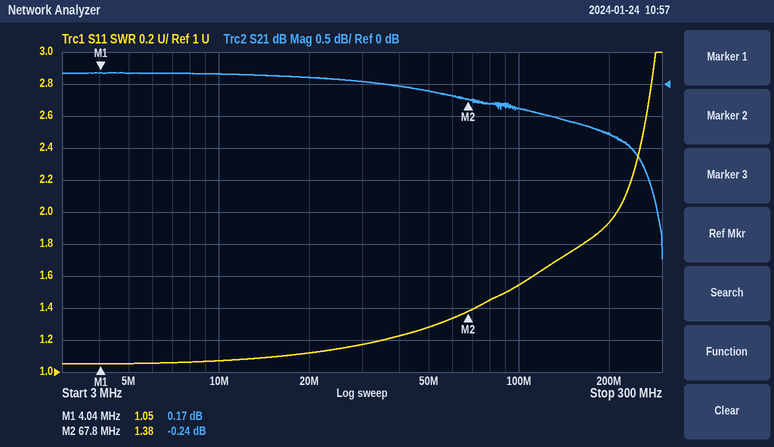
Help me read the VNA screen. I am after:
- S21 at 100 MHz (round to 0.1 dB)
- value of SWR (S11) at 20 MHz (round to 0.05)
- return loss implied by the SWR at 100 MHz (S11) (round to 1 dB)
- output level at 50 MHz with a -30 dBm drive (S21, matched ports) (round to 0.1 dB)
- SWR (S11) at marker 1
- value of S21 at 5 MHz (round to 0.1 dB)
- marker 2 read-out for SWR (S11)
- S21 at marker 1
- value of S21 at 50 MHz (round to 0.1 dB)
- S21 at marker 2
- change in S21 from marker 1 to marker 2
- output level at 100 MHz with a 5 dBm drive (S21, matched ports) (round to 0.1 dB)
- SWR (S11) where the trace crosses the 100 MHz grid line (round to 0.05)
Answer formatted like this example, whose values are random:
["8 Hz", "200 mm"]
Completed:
["-0.4 dB", "1.10", "13 dB", "-30.1 dBm", "1.05", "0.2 dB", "1.38", "0.17 dB", "-0.1 dB", "-0.24 dB", "-0.41 dB", "4.6 dBm", "1.55"]
